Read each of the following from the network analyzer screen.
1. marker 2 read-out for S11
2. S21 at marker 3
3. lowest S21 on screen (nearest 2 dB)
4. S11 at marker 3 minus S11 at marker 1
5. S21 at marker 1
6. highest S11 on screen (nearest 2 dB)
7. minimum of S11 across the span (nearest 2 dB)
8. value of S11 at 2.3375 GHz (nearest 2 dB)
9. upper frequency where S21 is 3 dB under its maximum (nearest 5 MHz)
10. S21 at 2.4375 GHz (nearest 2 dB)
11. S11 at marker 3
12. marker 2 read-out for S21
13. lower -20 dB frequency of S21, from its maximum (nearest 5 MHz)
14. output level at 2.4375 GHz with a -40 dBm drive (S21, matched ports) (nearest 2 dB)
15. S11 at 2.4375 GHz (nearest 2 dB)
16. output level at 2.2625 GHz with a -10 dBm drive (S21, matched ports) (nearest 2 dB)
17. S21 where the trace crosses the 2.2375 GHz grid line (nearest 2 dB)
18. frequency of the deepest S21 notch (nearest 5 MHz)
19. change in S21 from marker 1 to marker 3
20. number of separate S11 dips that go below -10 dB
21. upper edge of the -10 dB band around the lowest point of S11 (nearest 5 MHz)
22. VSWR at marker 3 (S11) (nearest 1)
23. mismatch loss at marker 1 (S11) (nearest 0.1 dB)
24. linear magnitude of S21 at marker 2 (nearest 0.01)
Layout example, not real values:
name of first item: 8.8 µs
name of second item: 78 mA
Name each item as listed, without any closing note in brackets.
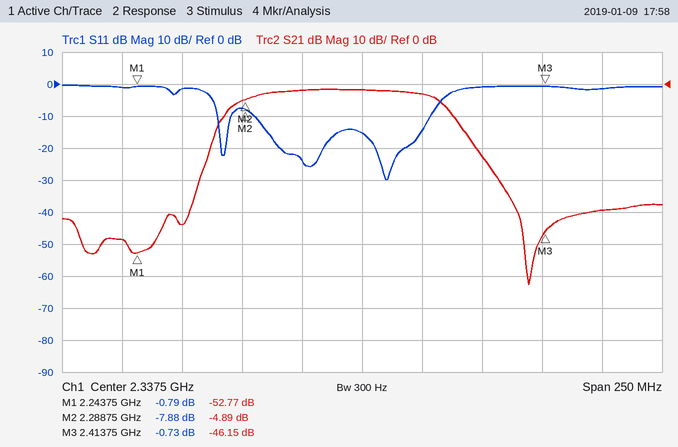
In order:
marker 2 read-out for S11: -7.88 dB
S21 at marker 3: -46.15 dB
lowest S21 on screen: -62 dB
S11 at marker 3 minus S11 at marker 1: 0.06 dB
S21 at marker 1: -52.77 dB
highest S11 on screen: 0 dB
minimum of S11 across the span: -30 dB
value of S11 at 2.3375 GHz: -16 dB
upper frequency where S21 is 3 dB under its maximum: 2.370 GHz
S21 at 2.4375 GHz: -40 dB
S11 at marker 3: -0.73 dB
marker 2 read-out for S21: -4.89 dB
lower -20 dB frequency of S21, from its maximum: 2.275 GHz
output level at 2.4375 GHz with a -40 dBm drive (S21, matched ports): -80 dBm
S11 at 2.4375 GHz: -2 dB
output level at 2.2625 GHz with a -10 dBm drive (S21, matched ports): -54 dBm
S21 where the trace crosses the 2.2375 GHz grid line: -48 dB
frequency of the deepest S21 notch: 2.405 GHz
change in S21 from marker 1 to marker 3: 6.62 dB
number of separate S11 dips that go below -10 dB: 3
upper edge of the -10 dB band around the lowest point of S11: 2.365 GHz
VSWR at marker 3 (S11): 24
mismatch loss at marker 1 (S11): 7.8 dB
linear magnitude of S21 at marker 2: 0.57
